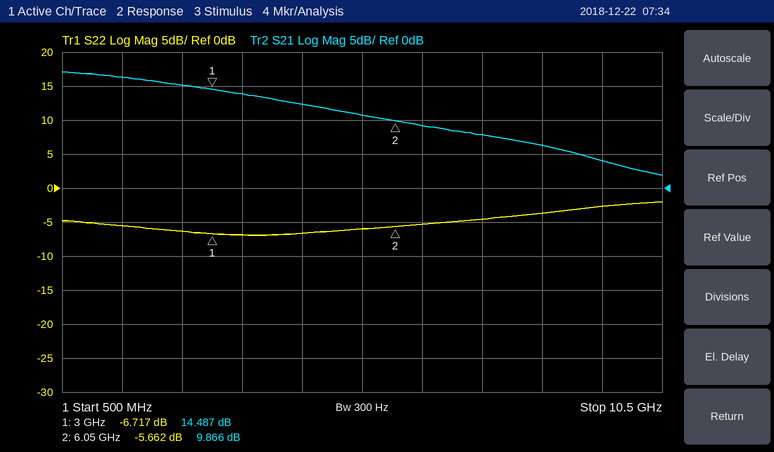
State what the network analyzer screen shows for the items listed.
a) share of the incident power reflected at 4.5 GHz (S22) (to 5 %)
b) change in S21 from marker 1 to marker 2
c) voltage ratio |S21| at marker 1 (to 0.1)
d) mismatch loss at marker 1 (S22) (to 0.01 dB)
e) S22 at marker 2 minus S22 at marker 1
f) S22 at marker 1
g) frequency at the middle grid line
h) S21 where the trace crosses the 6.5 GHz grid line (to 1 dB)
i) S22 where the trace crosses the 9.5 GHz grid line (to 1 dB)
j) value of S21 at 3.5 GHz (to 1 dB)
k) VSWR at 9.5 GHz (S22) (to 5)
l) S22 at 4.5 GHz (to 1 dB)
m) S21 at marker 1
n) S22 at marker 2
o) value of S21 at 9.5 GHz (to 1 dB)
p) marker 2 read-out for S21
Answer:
20 %
-4.621 dB
5.3
1.04 dB
1.055 dB
-6.717 dB
5.5 GHz
9 dB
-3 dB
14 dB
5
-7 dB
14.487 dB
-5.662 dB
4 dB
9.866 dB
